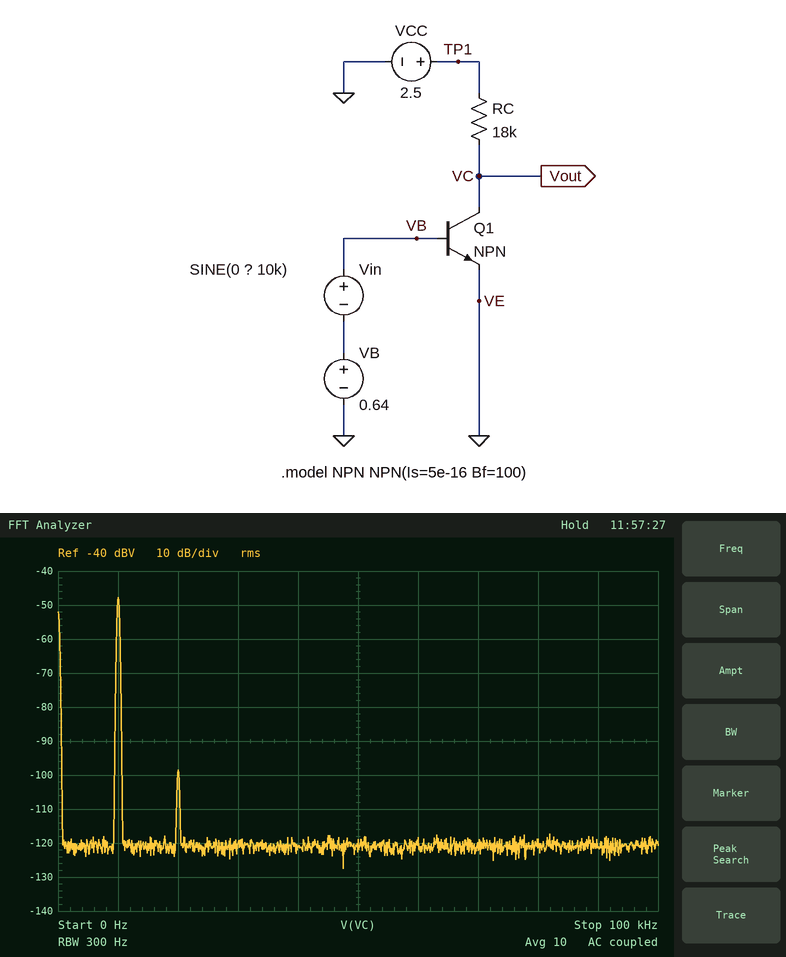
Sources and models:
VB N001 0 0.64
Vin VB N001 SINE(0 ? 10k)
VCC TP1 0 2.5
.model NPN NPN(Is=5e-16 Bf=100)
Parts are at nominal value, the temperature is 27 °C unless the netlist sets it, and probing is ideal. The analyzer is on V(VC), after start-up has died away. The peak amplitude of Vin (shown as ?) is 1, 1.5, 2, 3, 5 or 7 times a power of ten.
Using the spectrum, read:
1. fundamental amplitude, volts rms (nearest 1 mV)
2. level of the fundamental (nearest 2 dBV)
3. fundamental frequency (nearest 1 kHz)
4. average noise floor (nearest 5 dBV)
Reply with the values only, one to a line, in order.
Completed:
4 mV
-48 dBV
10 kHz
-120 dBV
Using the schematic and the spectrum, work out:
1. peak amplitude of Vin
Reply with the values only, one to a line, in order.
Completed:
300 µV
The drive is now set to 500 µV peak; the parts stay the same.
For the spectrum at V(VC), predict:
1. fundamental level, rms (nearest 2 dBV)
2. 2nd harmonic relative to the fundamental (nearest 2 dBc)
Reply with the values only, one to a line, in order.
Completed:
-44 dBV
-46 dBc
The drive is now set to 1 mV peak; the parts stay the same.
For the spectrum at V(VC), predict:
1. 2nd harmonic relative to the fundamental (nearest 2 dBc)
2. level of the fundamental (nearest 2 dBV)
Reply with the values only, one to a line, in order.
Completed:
-40 dBc
-38 dBV
